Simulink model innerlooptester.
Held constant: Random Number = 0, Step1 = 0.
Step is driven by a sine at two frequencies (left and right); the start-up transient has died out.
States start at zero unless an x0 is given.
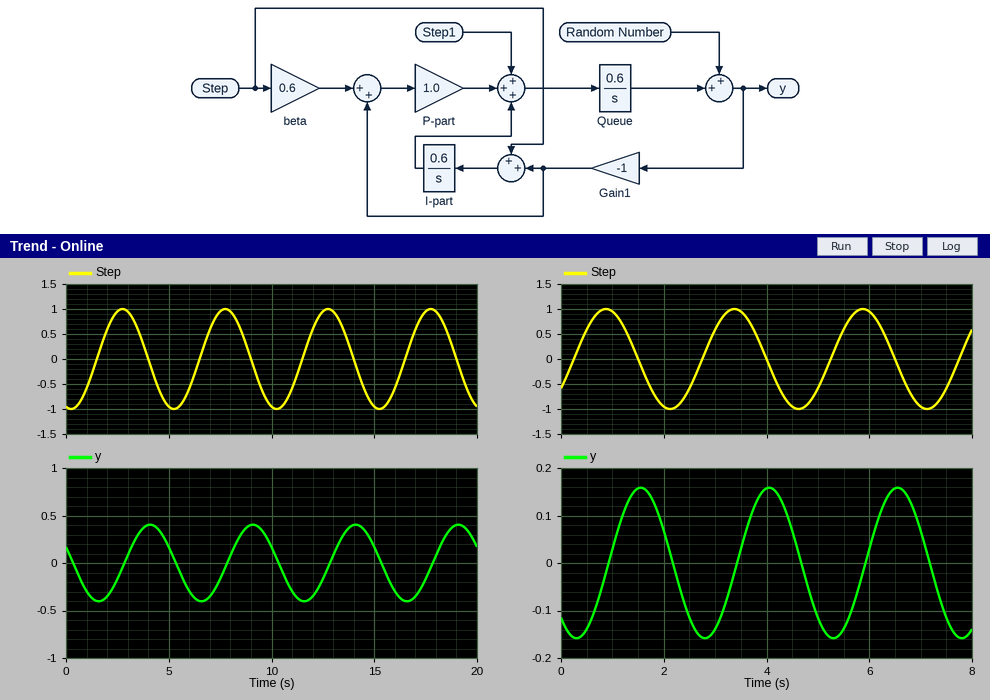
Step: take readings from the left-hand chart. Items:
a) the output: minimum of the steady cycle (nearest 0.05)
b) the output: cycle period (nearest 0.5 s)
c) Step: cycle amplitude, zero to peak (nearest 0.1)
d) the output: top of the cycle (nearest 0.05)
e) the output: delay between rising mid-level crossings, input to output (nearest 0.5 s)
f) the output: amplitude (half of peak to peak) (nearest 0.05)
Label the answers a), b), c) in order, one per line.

a) -0.40
b) 5.0 s
c) 1.0
d) 0.40
e) 1.5 s
f) 0.40
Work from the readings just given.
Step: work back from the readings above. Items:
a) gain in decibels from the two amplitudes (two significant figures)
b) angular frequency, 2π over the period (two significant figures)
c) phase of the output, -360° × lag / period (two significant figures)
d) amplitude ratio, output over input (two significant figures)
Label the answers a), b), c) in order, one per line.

a) -8.0 dB
b) 1.3 rad/s
c) -110°
d) 0.40
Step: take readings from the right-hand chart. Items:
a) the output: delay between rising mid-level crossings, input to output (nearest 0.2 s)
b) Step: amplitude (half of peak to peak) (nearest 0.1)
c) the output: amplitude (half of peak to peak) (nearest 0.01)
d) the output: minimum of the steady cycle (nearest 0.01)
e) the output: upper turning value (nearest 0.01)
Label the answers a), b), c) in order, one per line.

a) 0.6 s
b) 1.0
c) 0.16
d) -0.16
e) 0.16
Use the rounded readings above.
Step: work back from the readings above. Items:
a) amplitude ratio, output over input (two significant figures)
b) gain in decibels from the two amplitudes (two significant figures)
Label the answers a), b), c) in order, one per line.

a) 0.16
b) -16 dB
